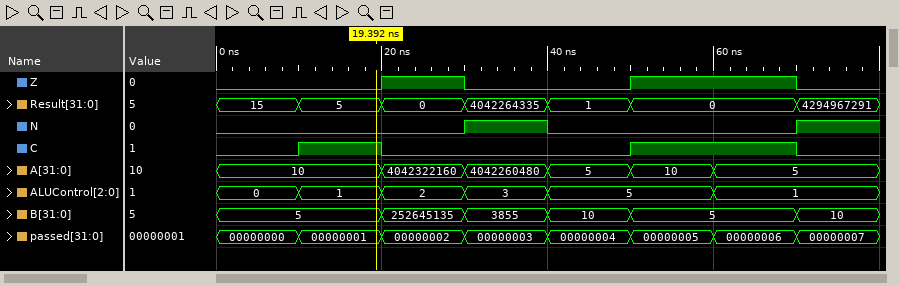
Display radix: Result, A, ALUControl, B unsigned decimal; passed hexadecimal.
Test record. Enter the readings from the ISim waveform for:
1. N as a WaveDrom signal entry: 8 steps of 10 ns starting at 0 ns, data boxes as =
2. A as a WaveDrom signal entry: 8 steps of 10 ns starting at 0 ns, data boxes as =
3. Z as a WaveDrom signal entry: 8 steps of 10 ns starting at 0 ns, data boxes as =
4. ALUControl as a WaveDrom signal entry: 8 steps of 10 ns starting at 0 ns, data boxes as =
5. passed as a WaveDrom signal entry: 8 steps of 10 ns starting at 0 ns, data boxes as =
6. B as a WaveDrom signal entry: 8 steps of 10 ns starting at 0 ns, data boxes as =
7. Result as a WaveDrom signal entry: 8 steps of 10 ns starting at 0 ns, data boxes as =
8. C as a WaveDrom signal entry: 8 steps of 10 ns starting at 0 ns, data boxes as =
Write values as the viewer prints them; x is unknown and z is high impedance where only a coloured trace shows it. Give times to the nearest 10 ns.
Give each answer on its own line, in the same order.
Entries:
{name: 'N', wave: '0..10..1'}
{name: 'A', wave: '=.=====.', data: '10 4042322160 4042260480 5 10 5'}
{name: 'Z', wave: '0.10.1.0'}
{name: 'ALUControl', wave: '=====.=.', data: '0 1 2 3 5 1'}
{name: 'passed', wave: '========', data: '00000000 00000001 00000002 00000003 00000004 00000005 00000006 00000007'}
{name: 'B', wave: '=.====.=', data: '5 252645135 3855 10 5 10'}
{name: 'Result', wave: '======.=', data: '15 5 0 4042264335 1 0 4294967291'}
{name: 'C', wave: '010..1.0'}
